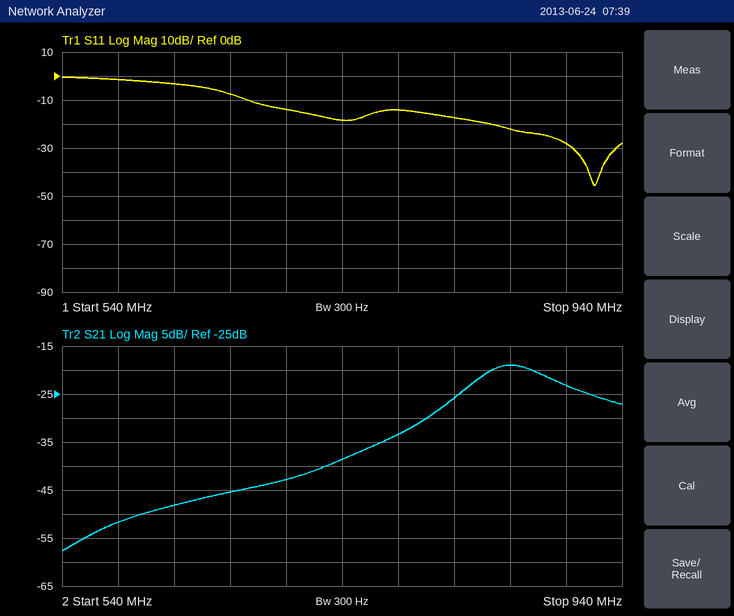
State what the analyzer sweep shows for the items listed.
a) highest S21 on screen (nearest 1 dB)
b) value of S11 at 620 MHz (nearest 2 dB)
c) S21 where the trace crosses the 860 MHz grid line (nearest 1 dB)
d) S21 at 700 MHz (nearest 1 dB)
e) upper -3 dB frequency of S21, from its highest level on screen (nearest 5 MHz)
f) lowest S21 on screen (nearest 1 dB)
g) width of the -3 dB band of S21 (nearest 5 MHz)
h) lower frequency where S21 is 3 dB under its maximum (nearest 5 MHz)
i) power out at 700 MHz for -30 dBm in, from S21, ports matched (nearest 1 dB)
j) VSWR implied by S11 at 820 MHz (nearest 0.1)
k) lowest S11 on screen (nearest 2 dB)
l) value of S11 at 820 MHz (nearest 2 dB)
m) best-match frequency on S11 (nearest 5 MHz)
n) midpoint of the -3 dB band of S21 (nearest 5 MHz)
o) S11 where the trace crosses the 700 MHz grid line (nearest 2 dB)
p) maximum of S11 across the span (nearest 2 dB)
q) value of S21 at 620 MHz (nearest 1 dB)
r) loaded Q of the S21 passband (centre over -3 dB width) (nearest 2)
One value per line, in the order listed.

-19 dB
-4 dB
-19 dB
-43 dB
890 MHz
-58 dB
55 MHz
835 MHz
-73 dBm
1.3
-46 dB
-18 dB
920 MHz
865 MHz
-14 dB
0 dB
-48 dB
16
